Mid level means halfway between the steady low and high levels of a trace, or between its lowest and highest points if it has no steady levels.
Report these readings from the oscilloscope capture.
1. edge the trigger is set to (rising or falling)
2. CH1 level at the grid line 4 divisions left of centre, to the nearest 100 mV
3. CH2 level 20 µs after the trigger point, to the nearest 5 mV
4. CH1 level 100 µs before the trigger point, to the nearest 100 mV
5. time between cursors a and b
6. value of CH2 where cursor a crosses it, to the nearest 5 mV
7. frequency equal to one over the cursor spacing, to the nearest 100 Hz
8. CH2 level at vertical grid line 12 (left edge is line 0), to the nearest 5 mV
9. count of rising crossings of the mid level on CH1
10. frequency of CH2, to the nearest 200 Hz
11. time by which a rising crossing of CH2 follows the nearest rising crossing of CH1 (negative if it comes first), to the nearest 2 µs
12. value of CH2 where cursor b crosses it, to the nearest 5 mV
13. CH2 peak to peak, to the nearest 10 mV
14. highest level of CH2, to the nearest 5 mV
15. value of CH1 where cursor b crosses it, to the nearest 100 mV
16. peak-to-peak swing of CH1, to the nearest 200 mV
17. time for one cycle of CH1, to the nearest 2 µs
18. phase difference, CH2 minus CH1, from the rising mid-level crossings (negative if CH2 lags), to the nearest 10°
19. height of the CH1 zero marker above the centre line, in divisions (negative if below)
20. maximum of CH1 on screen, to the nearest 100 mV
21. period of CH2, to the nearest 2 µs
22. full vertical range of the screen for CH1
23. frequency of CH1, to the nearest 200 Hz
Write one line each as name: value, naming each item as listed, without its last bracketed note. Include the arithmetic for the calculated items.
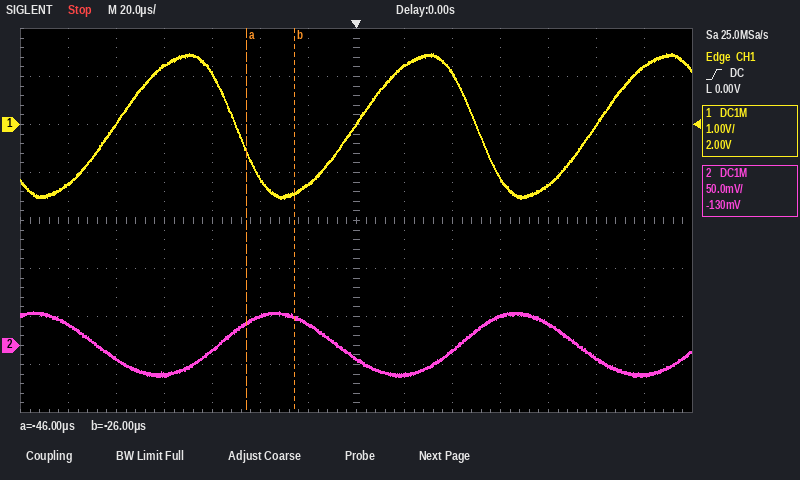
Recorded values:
edge the trigger is set to: rising
CH1 level at the grid line 4 divisions left of centre, to the nearest 100 mV: 1.2 V
CH2 level 20 µs after the trigger point, to the nearest 5 mV: -30 mV
CH1 level 100 µs before the trigger point, to the nearest 100 mV: 0.0 V
time between cursors a and b: -26 µs − (-46 µs) = 20 µs
value of CH2 where cursor a crosses it, to the nearest 5 mV: 25 mV
frequency equal to one over the cursor spacing, to the nearest 100 Hz: 1 / 20 µs ≈ 50.0 kHz
CH2 level at vertical grid line 12 (left edge is line 0), to the nearest 5 mV: -15 mV
count of rising crossings of the mid level on CH1: 3
frequency of CH2, to the nearest 200 Hz: 1 / 100 µs ≈ 10.0 kHz
time by which a rising crossing of CH2 follows the nearest rising crossing of CH1 (negative if it comes first), to the nearest 2 µs: +44 µs
value of CH2 where cursor b crosses it, to the nearest 5 mV: 30 mV
CH2 peak to peak, to the nearest 10 mV: 70 mV
highest level of CH2, to the nearest 5 mV: 35 mV
value of CH1 where cursor b crosses it, to the nearest 100 mV: -1.4 V
peak-to-peak swing of CH1, to the nearest 200 mV: 3.0 V
time for one cycle of CH1, to the nearest 2 µs: 100 µs
phase difference, CH2 minus CH1, from the rising mid-level crossings (negative if CH2 lags), to the nearest 10°: −360° × (+44 µs) / 100 µs ≈ -158°, so -160° to the nearest 10°
height of the CH1 zero marker above the centre line, in divisions: +2.0 div
maximum of CH1 on screen, to the nearest 100 mV: 1.5 V
period of CH2, to the nearest 2 µs: 100 µs
full vertical range of the screen for CH1: 8 V
frequency of CH1, to the nearest 200 Hz: 1 / 100 µs ≈ 10.0 kHz
